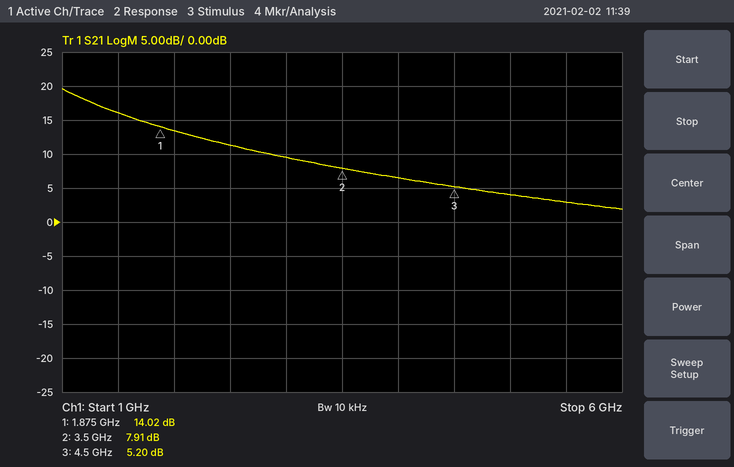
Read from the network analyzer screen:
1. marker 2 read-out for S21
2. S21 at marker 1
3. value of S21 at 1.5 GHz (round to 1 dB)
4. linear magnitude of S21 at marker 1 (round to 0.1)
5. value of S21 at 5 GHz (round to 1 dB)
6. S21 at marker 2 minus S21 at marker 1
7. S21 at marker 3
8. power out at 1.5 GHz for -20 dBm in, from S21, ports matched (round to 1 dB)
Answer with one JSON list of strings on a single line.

["7.91 dB", "14.02 dB", "16 dB", "5.0", "4 dB", "-6.11 dB", "5.20 dB", "-4 dBm"]
